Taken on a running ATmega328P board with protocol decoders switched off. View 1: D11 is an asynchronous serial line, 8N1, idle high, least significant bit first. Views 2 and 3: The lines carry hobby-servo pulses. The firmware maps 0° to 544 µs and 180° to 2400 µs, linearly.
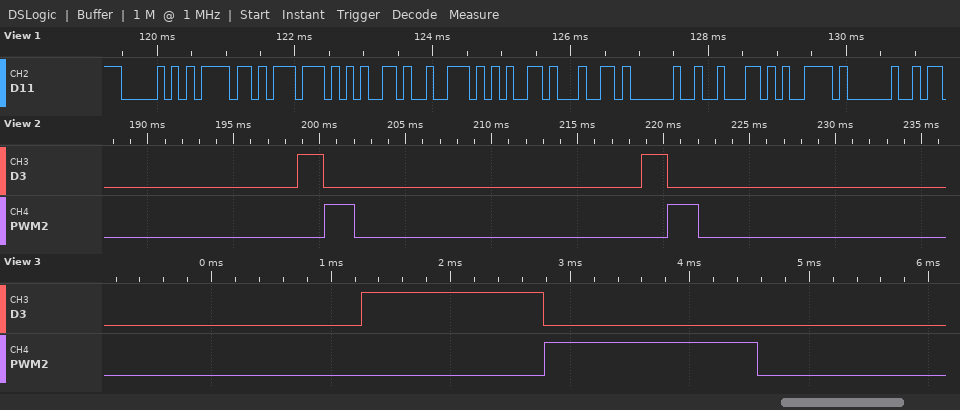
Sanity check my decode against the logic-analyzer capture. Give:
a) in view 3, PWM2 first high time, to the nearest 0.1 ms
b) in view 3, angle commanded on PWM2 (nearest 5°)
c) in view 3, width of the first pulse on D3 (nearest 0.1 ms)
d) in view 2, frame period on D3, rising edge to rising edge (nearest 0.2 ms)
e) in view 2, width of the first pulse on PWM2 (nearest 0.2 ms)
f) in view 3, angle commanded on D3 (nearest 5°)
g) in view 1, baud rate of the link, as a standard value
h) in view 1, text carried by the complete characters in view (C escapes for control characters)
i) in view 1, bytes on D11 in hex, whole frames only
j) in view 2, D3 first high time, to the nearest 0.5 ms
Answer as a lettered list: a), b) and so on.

a) 1.8 ms
b) 120°
c) 1.5 ms
d) 20.0 ms
e) 1.8 ms
f) 95°
g) 9600 baud
h) "Powered by "
i) 0x50 0x6F 0x77 0x65 0x72 0x65 0x64 0x20 0x62 0x79 0x20
j) 1.5 ms
